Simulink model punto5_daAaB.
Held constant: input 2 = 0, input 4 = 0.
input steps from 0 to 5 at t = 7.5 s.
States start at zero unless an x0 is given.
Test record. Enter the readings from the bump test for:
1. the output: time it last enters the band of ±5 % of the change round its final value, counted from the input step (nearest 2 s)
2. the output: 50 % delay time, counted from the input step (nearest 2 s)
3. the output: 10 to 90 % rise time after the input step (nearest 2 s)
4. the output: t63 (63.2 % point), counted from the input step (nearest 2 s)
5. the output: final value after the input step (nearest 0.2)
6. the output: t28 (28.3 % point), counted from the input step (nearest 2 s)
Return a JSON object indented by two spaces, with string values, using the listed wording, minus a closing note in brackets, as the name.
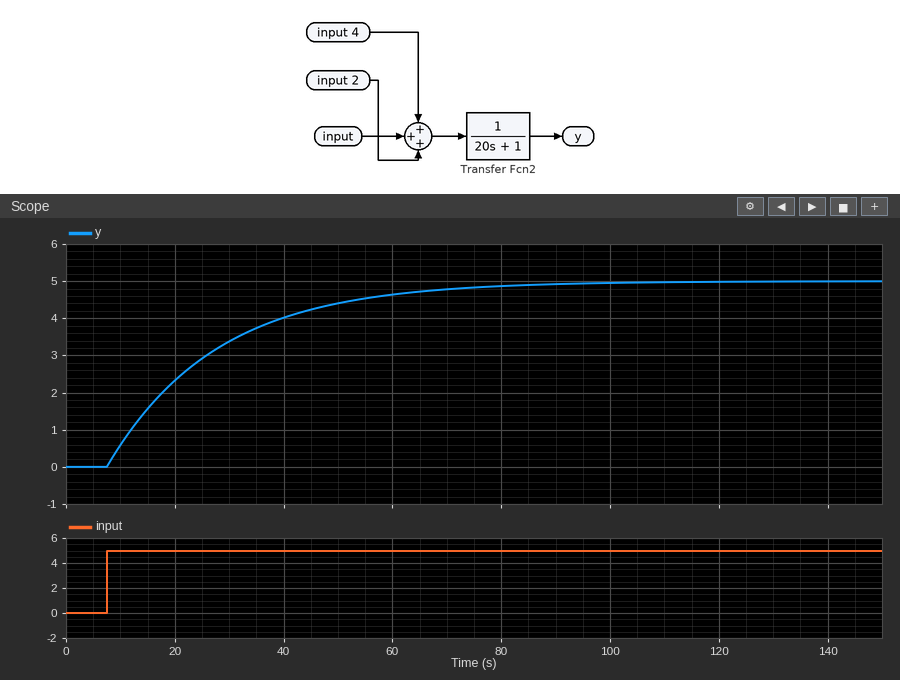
{
  "the output: time it last enters the band of ±5 % of the change round its final value, counted from the input step": "60 s",
  "the output: 50 % delay time, counted from the input step": "14 s",
  "the output: 10 to 90 % rise time after the input step": "44 s",
  "the output: t63 (63.2 % point), counted from the input step": "20 s",
  "the output: final value after the input step": "5.0",
  "the output: t28 (28.3 % point), counted from the input step": "6 s"
}
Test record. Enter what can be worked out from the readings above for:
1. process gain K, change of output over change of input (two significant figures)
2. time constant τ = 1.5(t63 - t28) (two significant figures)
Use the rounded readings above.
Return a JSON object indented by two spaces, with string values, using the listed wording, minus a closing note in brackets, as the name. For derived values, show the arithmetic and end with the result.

{
  "process gain K, change of output over change of input": "(5 - 0) / 5 = 1.0",
  "time constant τ = 1.5(t63 - t28)": "1.5 × (20 - 6) = 21 s"
}
